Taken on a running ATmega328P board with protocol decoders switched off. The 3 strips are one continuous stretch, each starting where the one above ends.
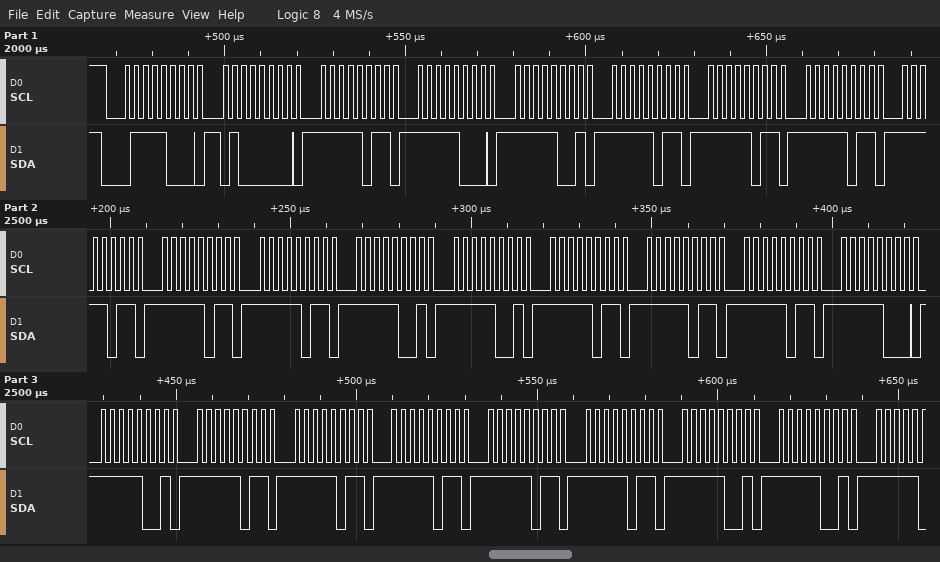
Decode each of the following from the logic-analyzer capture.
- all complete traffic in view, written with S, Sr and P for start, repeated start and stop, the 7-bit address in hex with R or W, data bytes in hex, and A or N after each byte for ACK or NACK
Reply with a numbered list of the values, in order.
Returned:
1. S 3CW A 40 A FB A F8 A F9 A FB A FB A FB A FB A FB A FB A F9 A F9 A FB A FB A FB A F8 A F9 A FB A FB A FB A FB A FB A F9 A F9 A
